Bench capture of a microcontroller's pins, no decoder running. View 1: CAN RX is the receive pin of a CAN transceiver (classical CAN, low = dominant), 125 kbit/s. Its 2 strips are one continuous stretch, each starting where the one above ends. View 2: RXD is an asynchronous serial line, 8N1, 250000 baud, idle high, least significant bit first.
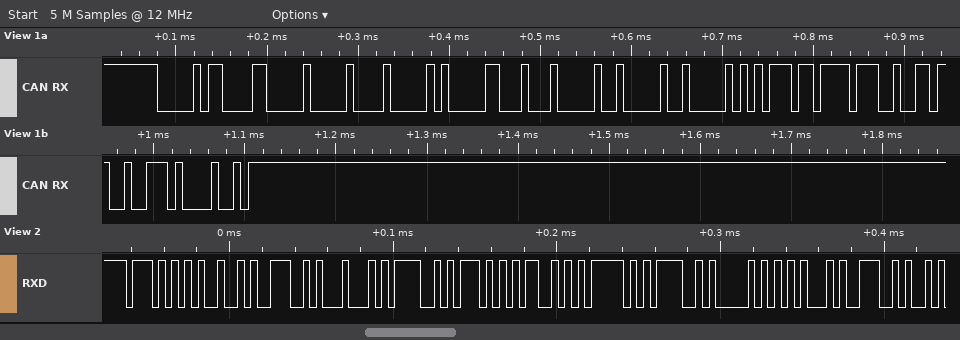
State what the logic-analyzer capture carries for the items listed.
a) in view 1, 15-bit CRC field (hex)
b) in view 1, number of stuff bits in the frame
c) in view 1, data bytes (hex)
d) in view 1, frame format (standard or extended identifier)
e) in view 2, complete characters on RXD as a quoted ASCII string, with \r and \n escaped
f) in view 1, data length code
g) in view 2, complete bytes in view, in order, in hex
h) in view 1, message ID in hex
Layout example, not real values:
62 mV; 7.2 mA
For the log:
0x4E84; 8; 22 20 20 20 57 6F 72 6C; extended; "WINDOWS_OPEN"; 8; 57 49 4E 44 4F 57 53 5F 4F 50 45 4E; 0x00C00008
